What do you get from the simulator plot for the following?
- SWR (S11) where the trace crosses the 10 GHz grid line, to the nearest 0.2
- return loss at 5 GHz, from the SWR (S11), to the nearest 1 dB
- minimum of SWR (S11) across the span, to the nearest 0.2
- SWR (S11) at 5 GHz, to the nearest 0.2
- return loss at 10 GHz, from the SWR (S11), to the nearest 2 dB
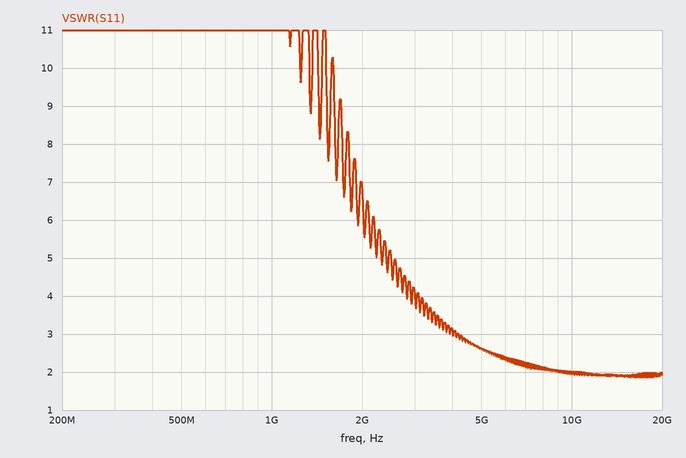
2.0
7 dB
1.8
2.6
10 dB
